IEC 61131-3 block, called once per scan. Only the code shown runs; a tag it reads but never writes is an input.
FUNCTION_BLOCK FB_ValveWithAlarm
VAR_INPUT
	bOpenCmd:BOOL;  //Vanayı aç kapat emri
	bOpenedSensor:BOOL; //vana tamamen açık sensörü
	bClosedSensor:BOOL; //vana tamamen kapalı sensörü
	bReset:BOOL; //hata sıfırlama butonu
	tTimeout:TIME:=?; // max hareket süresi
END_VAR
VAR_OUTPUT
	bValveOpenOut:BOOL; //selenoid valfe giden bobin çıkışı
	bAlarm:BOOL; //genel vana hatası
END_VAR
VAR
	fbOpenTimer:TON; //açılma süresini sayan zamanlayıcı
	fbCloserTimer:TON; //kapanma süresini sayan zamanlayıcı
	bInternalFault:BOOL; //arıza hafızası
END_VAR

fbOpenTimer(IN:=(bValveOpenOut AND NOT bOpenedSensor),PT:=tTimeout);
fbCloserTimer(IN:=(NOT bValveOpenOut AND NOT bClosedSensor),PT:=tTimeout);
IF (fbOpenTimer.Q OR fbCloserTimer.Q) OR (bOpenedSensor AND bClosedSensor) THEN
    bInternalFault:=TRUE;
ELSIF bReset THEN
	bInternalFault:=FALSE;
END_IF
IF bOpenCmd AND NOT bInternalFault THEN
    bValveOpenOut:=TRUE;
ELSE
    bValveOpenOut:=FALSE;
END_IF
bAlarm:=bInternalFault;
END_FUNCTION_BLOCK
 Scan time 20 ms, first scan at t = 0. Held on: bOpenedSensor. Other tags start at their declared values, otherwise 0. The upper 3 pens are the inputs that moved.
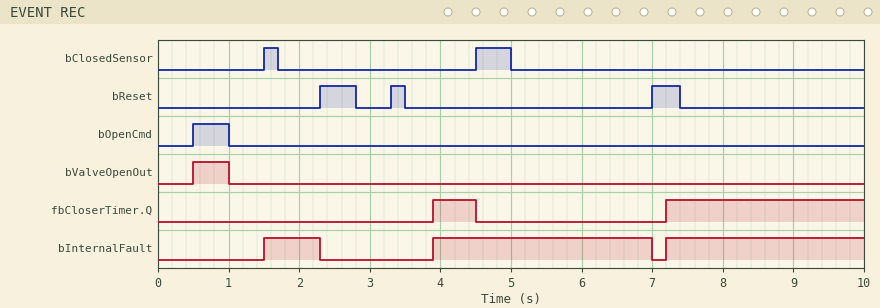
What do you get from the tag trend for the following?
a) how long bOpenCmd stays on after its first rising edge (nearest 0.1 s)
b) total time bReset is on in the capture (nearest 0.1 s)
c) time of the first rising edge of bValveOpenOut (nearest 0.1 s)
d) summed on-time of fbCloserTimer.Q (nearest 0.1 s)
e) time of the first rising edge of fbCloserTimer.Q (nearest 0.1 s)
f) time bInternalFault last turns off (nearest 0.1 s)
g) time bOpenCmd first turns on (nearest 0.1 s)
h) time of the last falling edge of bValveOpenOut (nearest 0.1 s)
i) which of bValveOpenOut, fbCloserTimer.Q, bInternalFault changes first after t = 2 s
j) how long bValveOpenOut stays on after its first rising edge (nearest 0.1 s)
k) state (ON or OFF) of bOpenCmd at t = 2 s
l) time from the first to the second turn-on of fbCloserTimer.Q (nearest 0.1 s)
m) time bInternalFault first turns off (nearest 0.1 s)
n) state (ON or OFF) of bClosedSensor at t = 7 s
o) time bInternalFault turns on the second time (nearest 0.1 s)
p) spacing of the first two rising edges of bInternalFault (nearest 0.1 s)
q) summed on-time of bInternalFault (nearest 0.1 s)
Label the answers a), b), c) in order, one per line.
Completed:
a) 0.5 s
b) 1.1 s
c) 0.5 s
d) 3.4 s
e) 3.9 s
f) 7.0 s
g) 0.5 s
h) 1.0 s
i) bInternalFault
j) 0.5 s
k) OFF
l) 3.3 s
m) 2.3 s
n) OFF
o) 3.9 s
p) 2.4 s
q) 6.7 s
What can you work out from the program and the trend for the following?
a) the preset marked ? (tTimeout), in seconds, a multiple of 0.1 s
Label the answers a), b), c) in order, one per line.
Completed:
a) 2.2 s
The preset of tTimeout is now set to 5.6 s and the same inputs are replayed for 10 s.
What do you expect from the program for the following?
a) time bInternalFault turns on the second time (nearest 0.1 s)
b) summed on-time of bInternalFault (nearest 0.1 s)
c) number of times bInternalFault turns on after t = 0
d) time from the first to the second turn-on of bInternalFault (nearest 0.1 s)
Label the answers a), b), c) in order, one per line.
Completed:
a) 4.5 s
b) 3.3 s
c) 2
d) 3.0 s
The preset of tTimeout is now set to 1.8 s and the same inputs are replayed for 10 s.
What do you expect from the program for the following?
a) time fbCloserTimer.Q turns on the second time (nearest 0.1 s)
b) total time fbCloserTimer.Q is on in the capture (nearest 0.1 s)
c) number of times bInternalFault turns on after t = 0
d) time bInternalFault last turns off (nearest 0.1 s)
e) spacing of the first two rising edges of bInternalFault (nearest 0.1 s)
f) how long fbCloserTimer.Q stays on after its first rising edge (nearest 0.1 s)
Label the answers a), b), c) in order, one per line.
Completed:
a) 6.8 s
b) 4.2 s
c) 2
d) 2.3 s
e) 2.0 s
f) 1.0 s
